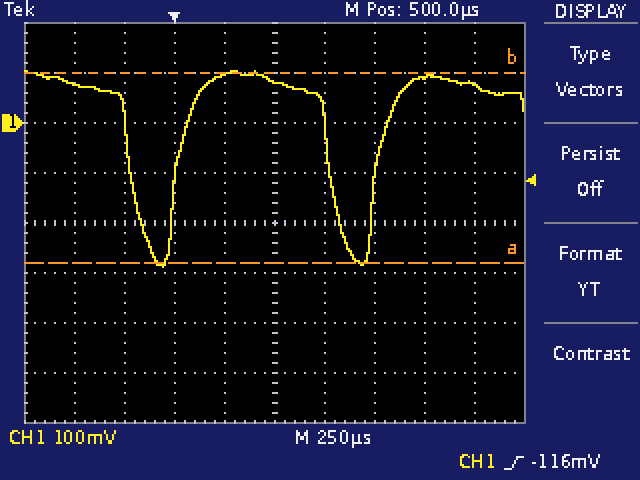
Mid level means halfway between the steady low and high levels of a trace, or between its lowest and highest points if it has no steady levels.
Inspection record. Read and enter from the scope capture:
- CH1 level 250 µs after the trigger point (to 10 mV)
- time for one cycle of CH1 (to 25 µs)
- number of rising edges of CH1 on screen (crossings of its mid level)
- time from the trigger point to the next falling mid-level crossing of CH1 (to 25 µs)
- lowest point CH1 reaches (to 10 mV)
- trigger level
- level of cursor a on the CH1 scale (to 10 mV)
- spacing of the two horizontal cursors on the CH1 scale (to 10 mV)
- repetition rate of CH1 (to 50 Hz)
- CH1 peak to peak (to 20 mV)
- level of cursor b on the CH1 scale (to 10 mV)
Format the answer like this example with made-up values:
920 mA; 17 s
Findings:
100 mV; 1.000 ms; 2; 775 µs; -290 mV; -116 mV; -280 mV; 380 mV; 1.00 kHz; 400 mV; 100 mV
